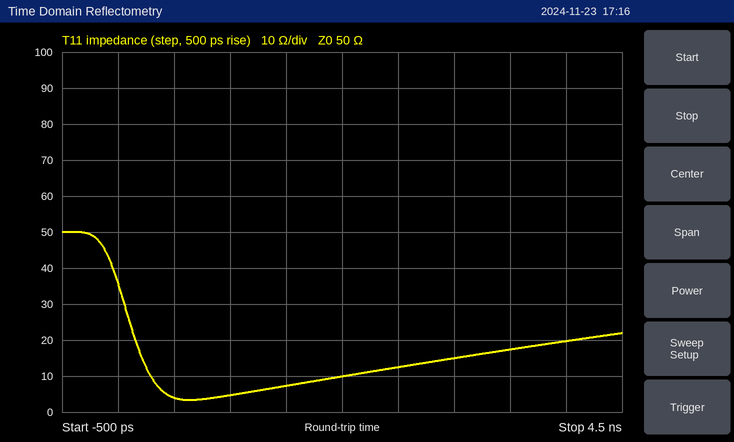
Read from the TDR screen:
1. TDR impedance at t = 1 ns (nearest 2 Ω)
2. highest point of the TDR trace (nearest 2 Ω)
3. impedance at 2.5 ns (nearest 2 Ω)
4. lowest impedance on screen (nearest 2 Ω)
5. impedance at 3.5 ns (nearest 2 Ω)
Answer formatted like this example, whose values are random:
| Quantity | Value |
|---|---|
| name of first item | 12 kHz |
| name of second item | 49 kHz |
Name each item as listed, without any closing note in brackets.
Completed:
| Quantity | Value |
|---|---|
| TDR impedance at t = 1 ns | 4 Ω |
| highest point of the TDR trace | 50 Ω |
| impedance at 2.5 ns | 12 Ω |
| lowest impedance on screen | 4 Ω |
| impedance at 3.5 ns | 18 Ω |
